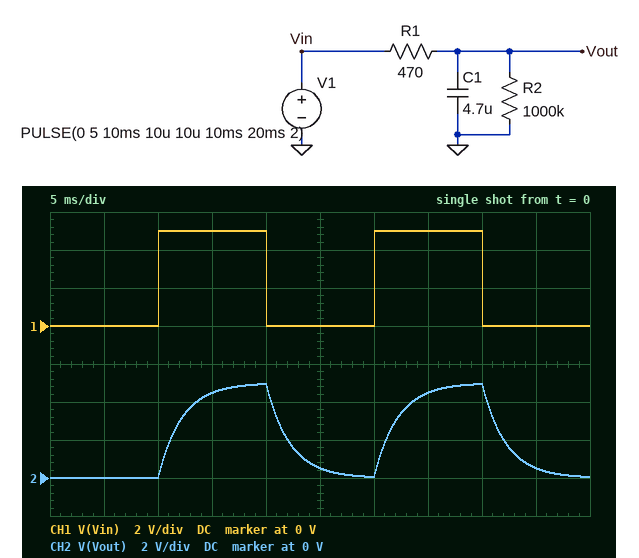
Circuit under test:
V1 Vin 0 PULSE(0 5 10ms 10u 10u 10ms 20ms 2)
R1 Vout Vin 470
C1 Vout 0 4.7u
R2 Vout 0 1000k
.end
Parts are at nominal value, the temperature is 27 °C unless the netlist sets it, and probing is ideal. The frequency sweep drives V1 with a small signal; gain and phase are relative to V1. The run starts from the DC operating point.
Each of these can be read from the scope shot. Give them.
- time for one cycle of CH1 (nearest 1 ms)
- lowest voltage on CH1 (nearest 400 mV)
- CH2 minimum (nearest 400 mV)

20 ms
0 V
0 V
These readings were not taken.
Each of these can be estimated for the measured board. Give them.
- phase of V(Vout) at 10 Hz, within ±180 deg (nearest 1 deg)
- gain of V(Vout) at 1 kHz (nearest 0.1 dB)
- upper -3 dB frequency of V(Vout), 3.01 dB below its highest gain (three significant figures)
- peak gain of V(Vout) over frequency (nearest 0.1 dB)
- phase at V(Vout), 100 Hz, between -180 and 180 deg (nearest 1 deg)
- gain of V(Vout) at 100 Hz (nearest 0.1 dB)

-8 deg
-22.9 dB
72.1 Hz
0 dB
-54 deg
-4.7 dB
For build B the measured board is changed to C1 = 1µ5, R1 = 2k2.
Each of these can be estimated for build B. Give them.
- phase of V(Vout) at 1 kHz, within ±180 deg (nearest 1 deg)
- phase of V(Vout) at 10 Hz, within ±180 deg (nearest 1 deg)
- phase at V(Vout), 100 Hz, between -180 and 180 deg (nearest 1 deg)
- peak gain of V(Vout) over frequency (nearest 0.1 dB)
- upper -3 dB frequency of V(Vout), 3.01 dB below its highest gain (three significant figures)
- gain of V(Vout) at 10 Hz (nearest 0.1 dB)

-87 deg
-12 deg
-64 deg
0 dB
48.3 Hz
-0.2 dB
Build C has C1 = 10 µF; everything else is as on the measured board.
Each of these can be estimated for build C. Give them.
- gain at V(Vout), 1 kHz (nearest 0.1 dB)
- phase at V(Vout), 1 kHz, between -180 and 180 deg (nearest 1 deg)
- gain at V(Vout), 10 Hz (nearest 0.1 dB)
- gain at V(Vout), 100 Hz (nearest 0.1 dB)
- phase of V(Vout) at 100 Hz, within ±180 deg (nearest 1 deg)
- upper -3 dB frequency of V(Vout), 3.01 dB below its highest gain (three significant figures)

-29.4 dB
-88 deg
-0.4 dB
-9.9 dB
-71 deg
33.9 Hz
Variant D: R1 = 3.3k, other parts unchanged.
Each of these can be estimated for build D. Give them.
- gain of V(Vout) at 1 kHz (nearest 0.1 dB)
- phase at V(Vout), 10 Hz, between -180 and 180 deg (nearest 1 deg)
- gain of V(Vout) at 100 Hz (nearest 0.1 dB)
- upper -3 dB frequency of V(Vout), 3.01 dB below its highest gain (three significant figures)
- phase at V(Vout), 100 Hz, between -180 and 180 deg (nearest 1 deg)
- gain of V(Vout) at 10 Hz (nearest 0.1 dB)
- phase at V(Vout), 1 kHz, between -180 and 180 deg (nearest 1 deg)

-39.8 dB
-44 deg
-19.8 dB
10.3 Hz
-84 deg
-2.9 dB
-89 deg
